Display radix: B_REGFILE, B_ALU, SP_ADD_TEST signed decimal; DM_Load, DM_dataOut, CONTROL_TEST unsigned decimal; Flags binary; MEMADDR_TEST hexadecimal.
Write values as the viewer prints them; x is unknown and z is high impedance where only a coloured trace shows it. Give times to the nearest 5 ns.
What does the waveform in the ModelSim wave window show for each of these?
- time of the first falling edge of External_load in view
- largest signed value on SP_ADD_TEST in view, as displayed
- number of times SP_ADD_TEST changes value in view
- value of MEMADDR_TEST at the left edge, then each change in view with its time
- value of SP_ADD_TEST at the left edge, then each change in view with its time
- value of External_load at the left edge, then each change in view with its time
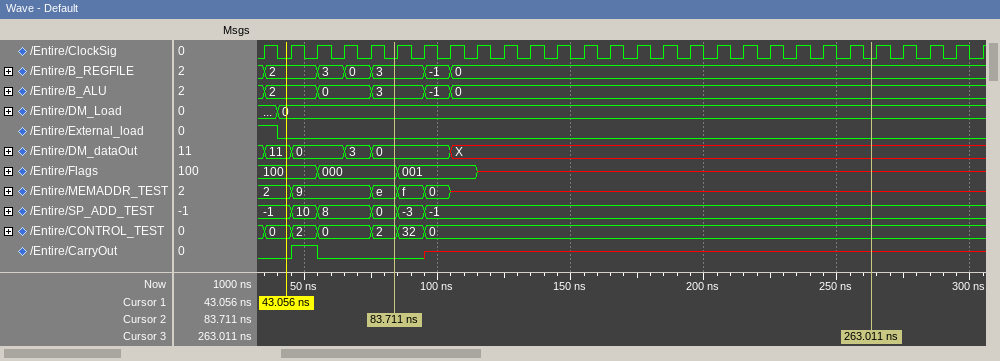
40 ns
10
5
2, 9 at 45 ns, e at 75 ns, f at 85 ns, 0 at 95 ns, x at 105 ns
-1, 10 at 45 ns, 8 at 55 ns, 0 at 75 ns, -3 at 85 ns, -1 at 95 ns
1, 0 at 40 ns
